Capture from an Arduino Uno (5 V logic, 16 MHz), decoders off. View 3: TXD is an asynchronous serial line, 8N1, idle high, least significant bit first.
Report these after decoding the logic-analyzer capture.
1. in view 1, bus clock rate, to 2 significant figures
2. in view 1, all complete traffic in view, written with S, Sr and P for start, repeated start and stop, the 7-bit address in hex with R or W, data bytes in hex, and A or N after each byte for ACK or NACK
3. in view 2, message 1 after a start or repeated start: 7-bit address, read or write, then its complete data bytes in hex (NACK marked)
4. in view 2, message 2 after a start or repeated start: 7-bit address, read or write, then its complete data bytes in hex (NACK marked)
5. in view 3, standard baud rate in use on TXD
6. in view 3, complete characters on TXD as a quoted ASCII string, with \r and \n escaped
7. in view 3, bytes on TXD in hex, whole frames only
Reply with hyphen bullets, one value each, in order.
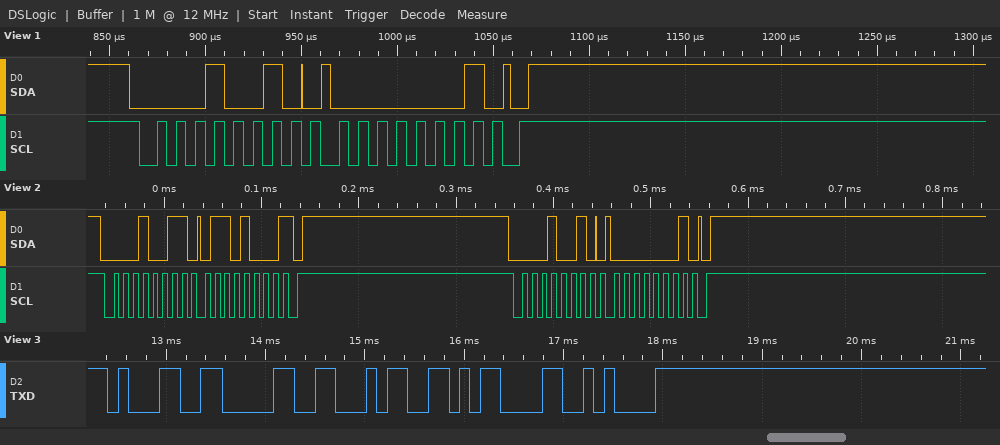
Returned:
- 100 kHz
- S 09W A 01 A P
- 0x09 read: 68 NACK
- 0x09 write: 01
- 9600 baud
- "104\r\n"
- 0x31 0x30 0x34 0x0D 0x0A
